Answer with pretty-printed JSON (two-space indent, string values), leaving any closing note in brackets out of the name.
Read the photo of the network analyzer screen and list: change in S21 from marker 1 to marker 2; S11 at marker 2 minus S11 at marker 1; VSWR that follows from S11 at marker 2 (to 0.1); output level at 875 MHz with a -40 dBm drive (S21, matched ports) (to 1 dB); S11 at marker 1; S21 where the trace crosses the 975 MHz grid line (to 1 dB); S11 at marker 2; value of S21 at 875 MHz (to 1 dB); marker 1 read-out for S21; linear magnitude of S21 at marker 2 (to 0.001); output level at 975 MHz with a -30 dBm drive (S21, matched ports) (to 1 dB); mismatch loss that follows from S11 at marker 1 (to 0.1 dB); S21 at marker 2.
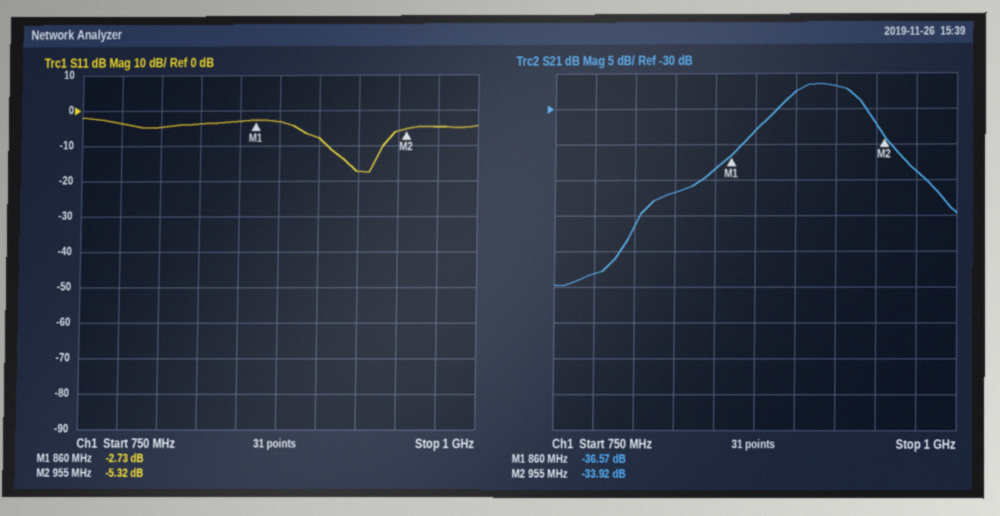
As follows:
{
  "change in S21 from marker 1 to marker 2": "2.65 dB",
  "S11 at marker 2 minus S11 at marker 1": "-2.59 dB",
  "VSWR that follows from S11 at marker 2": "3.4",
  "output level at 875 MHz with a -40 dBm drive (S21, matched ports)": "-73 dBm",
  "S11 at marker 1": "-2.73 dB",
  "S21 where the trace crosses the 975 MHz grid line": "-39 dB",
  "S11 at marker 2": "-5.32 dB",
  "value of S21 at 875 MHz": "-33 dB",
  "marker 1 read-out for S21": "-36.57 dB",
  "linear magnitude of S21 at marker 2": "0.020",
  "output level at 975 MHz with a -30 dBm drive (S21, matched ports)": "-69 dBm",
  "mismatch loss that follows from S11 at marker 1": "3.3 dB",
  "S21 at marker 2": "-33.92 dB"
}
